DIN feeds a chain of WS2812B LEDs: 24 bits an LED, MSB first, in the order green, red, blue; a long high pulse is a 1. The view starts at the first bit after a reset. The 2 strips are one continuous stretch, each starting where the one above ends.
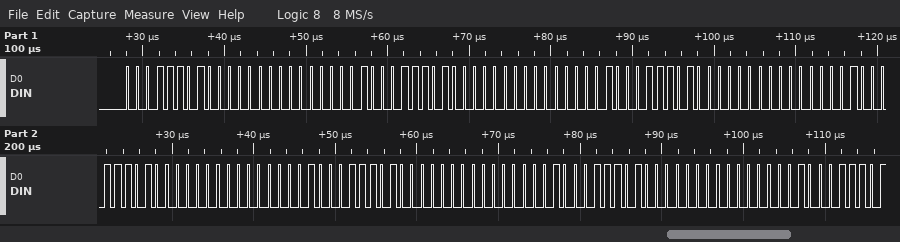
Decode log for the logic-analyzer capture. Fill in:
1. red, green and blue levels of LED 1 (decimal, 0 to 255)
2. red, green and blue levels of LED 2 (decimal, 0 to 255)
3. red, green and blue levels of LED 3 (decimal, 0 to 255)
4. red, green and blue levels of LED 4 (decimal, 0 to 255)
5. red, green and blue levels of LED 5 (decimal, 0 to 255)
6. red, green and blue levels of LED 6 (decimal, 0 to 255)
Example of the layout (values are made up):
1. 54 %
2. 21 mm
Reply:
1. 0, 29, 1
2. 0, 29, 1
3. 0, 29, 1
4. 0, 29, 1
5. 0, 29, 1
6. 0, 29, 1
